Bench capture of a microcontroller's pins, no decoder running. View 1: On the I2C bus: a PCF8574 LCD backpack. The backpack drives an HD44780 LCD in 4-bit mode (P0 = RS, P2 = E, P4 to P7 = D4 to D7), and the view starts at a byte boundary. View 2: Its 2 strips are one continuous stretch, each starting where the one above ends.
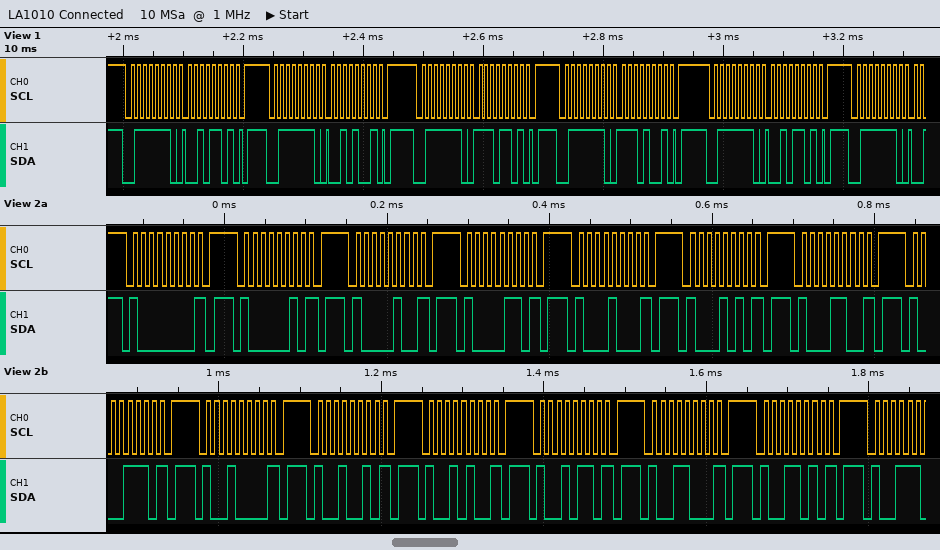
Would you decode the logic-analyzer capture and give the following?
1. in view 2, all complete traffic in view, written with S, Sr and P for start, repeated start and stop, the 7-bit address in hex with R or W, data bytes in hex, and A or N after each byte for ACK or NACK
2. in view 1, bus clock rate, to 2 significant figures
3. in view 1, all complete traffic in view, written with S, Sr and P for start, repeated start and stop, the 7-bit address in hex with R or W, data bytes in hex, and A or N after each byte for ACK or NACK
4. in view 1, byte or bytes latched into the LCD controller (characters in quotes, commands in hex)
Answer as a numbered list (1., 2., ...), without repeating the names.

1. S 40W N P S 41W N P S 42W N P S 43W N P S 44W N P S 45W N P S 46W N P S 47W N P S 48W N P S 49W N P S 4AW N P S 4BW N P S 4CW N P S 4DW N P
2. 100 kHz
3. S 3FW A 2D A P S 3FW A 29 A P S 3FW A ED A P S 3FW A E9 A P S 3FW A 2D A P S 3FW A
4. '.'
